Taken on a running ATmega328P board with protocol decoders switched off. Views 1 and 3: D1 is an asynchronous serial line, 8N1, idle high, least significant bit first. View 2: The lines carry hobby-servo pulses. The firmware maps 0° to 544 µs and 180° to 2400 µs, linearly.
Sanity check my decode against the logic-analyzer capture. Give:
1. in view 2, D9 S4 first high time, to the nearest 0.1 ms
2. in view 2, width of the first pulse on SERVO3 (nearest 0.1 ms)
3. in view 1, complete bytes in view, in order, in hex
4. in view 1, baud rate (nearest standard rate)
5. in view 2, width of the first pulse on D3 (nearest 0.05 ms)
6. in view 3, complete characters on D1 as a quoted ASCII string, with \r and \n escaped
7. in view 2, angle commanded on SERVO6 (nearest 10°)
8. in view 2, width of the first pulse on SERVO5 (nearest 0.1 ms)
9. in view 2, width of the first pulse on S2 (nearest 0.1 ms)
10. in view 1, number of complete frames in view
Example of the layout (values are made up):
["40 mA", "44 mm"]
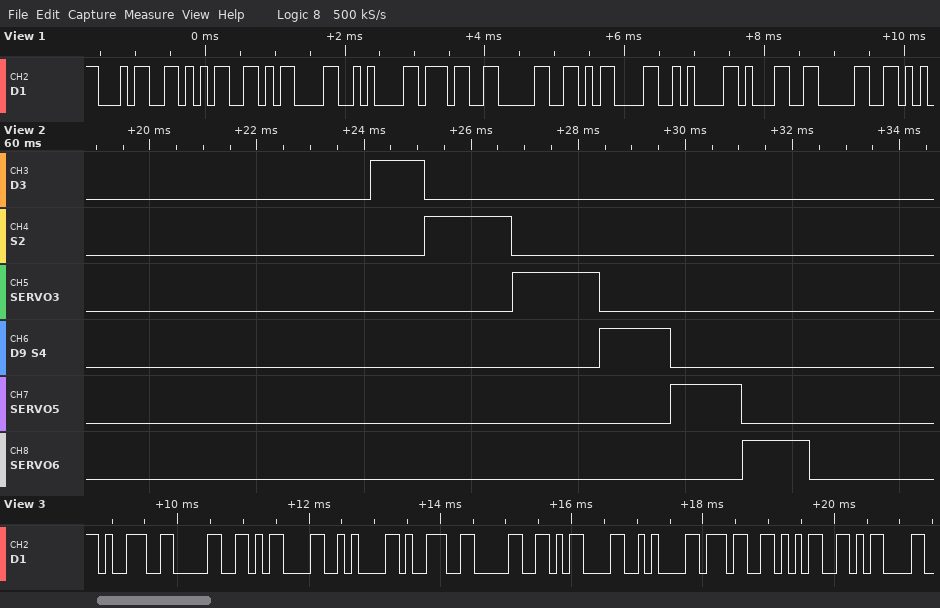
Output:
["1.3 ms", "1.6 ms", "34 35 0D 0A 37 30 0D 0A 31 30", "9600 baud", "1.00 ms", "\"90\\r\\n90\\r\\n75\\r\"", "70°", "1.3 ms", "1.6 ms", "10"]
